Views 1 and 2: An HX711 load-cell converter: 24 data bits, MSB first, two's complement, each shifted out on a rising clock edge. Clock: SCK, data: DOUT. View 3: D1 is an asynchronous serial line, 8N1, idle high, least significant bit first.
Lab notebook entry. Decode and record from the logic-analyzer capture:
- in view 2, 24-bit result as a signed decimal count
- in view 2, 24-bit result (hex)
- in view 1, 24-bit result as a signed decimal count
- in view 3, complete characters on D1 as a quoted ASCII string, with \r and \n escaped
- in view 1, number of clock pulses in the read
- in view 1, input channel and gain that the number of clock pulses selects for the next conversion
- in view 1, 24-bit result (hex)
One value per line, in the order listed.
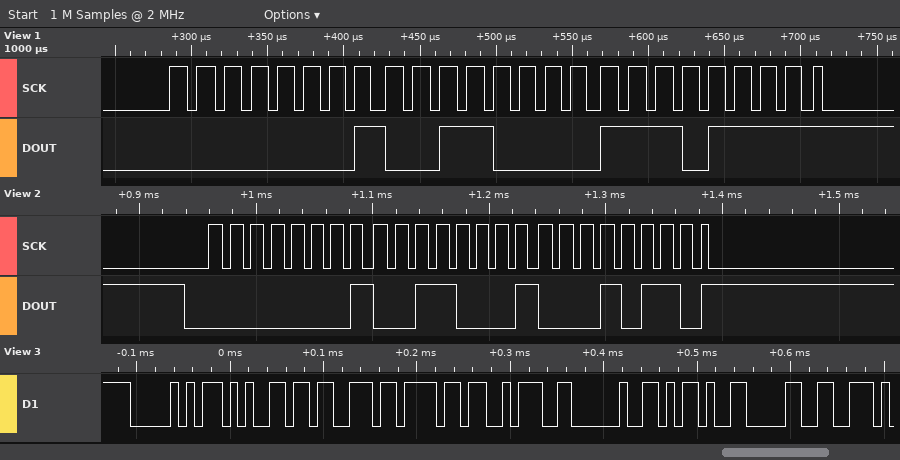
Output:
78102
0x013116
78063
"Peso: -0"
25
channel A, gain 128
0x0130EF
